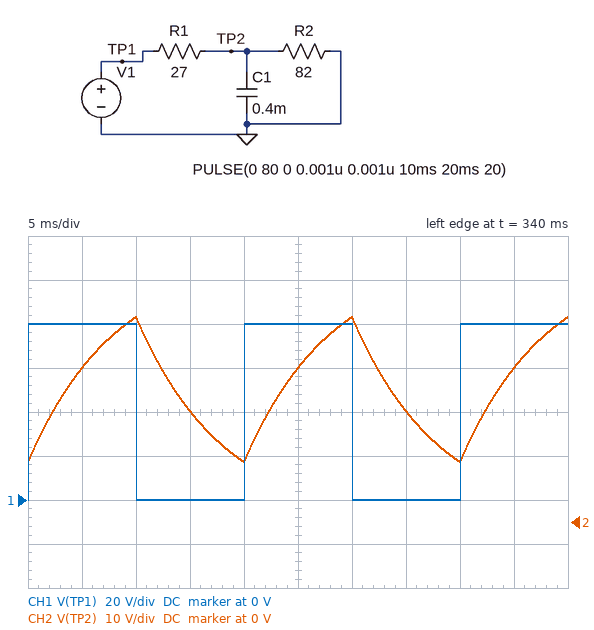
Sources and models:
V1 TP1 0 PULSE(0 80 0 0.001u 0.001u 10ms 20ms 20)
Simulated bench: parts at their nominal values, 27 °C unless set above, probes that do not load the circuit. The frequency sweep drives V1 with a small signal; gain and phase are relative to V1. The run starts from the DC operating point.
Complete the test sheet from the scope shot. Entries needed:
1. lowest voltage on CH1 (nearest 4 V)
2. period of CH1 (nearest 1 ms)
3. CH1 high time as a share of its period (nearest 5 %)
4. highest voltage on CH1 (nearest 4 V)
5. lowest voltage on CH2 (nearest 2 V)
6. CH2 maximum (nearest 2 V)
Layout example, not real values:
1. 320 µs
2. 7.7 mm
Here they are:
1. 0 V
2. 20 ms
3. 50 %
4. 80 V
5. 14 V
6. 46 V
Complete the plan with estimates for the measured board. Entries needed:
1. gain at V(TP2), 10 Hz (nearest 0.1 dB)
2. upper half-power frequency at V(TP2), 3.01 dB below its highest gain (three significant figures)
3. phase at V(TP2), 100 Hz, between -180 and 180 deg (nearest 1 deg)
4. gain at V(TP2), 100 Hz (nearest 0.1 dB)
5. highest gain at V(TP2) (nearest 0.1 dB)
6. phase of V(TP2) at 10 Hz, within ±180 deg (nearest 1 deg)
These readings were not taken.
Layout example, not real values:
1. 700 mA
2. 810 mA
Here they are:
1. -3.5 dB
2. 19.6 Hz
3. -79 deg
4. -16.8 dB
5. -2.5 dB
6. -27 deg
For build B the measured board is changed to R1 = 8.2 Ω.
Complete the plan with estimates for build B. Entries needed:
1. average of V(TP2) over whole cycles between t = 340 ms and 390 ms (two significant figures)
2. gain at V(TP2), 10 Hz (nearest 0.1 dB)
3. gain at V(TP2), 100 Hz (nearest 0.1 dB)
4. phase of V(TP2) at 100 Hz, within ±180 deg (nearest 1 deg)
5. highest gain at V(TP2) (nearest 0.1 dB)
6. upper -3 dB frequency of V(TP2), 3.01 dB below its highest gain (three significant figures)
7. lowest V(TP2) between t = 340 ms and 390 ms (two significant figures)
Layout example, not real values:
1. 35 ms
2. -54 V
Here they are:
1. 36 V
2. -1.0 dB
3. -7.4 dB
4. -62 deg
5. -0.8 dB
6. 53.4 Hz
7. 2.5 V
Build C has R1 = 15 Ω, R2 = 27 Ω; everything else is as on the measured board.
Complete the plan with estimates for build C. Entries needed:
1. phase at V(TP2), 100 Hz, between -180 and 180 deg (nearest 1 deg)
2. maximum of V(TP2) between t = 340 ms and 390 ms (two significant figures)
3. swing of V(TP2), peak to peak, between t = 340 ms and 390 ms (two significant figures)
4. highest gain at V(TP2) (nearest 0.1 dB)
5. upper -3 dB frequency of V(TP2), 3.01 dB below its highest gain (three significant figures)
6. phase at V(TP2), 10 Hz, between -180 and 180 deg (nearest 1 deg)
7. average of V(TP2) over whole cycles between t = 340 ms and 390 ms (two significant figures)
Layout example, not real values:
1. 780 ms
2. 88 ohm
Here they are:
1. -68 deg
2. 48 V
3. 44 V
4. -3.8 dB
5. 41.3 Hz
6. -14 deg
7. 26 V
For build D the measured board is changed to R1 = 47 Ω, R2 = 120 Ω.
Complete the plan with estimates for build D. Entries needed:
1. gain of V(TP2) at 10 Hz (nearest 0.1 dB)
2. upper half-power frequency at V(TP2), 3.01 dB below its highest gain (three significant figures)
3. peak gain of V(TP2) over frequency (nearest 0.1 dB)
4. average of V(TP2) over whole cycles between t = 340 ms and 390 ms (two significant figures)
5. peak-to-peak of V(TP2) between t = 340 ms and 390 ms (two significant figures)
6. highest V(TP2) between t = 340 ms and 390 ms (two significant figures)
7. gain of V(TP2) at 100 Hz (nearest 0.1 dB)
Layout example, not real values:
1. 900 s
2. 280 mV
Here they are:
1. -5.2 dB
2. 11.8 Hz
3. -2.9 dB
4. 29 V
5. 20 V
6. 39 V
7. -21.5 dB
